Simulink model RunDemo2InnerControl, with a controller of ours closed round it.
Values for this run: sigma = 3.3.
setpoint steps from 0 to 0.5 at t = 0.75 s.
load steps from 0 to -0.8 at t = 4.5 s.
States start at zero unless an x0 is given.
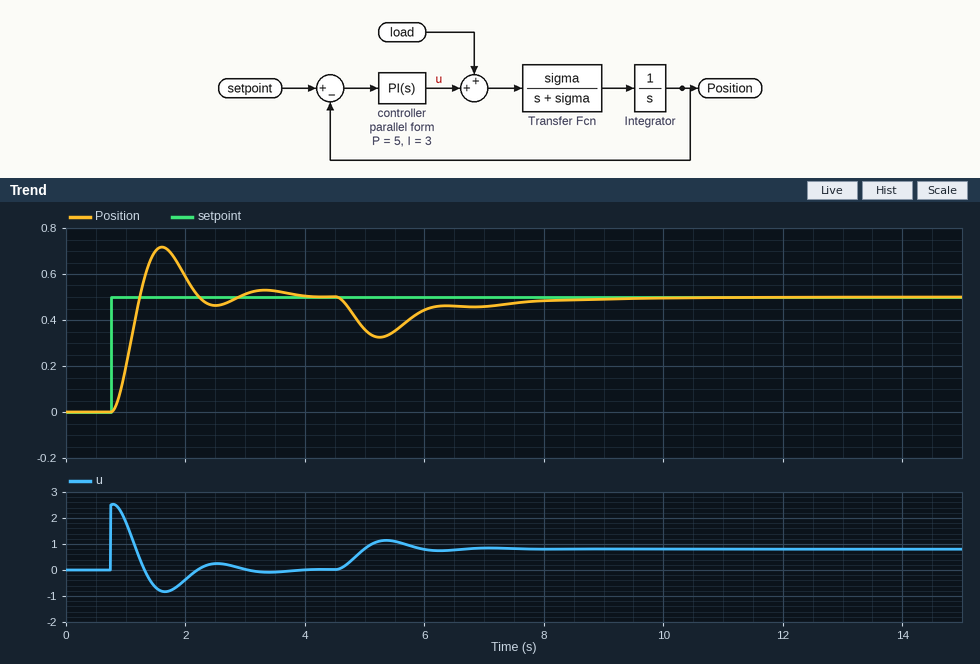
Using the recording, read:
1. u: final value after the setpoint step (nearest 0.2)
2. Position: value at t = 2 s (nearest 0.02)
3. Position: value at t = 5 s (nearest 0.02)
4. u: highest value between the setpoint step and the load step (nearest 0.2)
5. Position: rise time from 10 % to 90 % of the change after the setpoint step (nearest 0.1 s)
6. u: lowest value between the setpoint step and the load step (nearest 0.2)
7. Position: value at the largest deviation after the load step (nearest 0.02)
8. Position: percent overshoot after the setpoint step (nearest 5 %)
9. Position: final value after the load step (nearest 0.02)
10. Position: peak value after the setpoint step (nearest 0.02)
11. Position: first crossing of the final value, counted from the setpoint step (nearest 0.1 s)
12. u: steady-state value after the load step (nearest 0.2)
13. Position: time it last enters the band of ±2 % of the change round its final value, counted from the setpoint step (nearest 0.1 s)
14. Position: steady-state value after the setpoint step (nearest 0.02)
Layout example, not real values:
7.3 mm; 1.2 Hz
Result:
0.0; 0.58; 0.36; 2.6; 0.3 s; -0.8; 0.32; 45 %; 0.50; 0.72; 0.5 s; 0.8; 3.1 s; 0.50
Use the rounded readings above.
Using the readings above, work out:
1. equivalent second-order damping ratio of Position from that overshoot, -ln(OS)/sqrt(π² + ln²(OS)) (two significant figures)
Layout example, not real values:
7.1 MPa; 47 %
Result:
0.25
